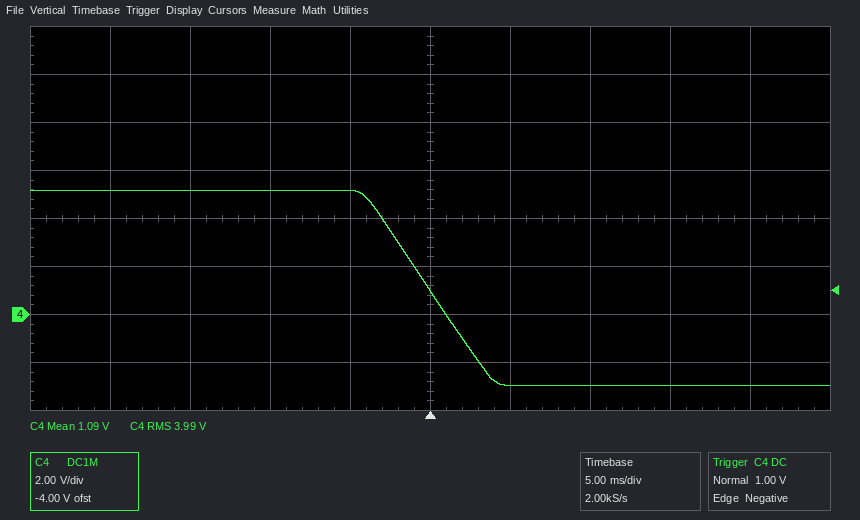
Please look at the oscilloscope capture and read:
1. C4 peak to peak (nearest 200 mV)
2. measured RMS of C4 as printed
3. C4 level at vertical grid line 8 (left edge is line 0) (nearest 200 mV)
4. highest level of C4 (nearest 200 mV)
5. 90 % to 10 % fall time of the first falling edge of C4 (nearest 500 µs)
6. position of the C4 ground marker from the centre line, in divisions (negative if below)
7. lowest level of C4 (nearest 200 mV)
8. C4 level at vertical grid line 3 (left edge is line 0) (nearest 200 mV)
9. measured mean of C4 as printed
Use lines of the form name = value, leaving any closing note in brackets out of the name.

C4 peak to peak = 8.2 V
measured RMS of C4 as printed = 3.99 V
C4 level at vertical grid line 8 (left edge is line 0) = -3.0 V
highest level of C4 = 5.2 V
90 % to 10 % fall time of the first falling edge of C4 = 6.5 ms
position of the C4 ground marker from the centre line, in divisions = -2.0 div
lowest level of C4 = -3.0 V
C4 level at vertical grid line 3 (left edge is line 0) = 5.2 V
measured mean of C4 as printed = 1.09 V
